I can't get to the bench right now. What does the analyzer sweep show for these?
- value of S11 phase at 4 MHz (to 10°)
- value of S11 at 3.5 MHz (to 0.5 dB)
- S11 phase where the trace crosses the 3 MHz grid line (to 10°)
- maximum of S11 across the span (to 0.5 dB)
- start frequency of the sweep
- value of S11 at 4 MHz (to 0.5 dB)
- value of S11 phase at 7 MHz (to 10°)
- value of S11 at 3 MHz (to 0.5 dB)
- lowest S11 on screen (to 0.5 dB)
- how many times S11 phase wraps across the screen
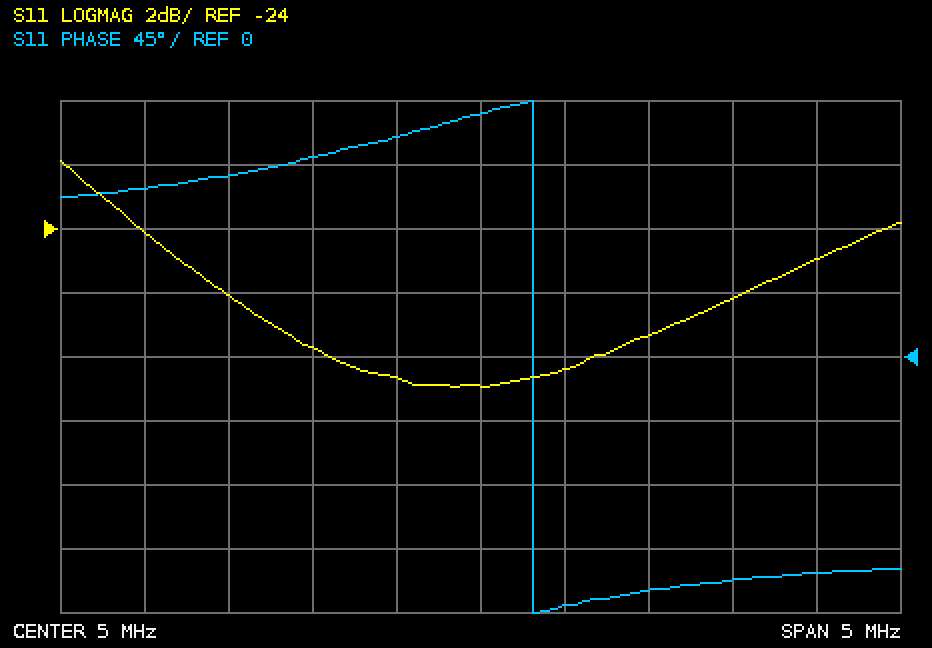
140°
-26.0 dB
120°
-22.0 dB
2.5 MHz
-27.5 dB
-150°
-24.0 dB
-29.0 dB
1
